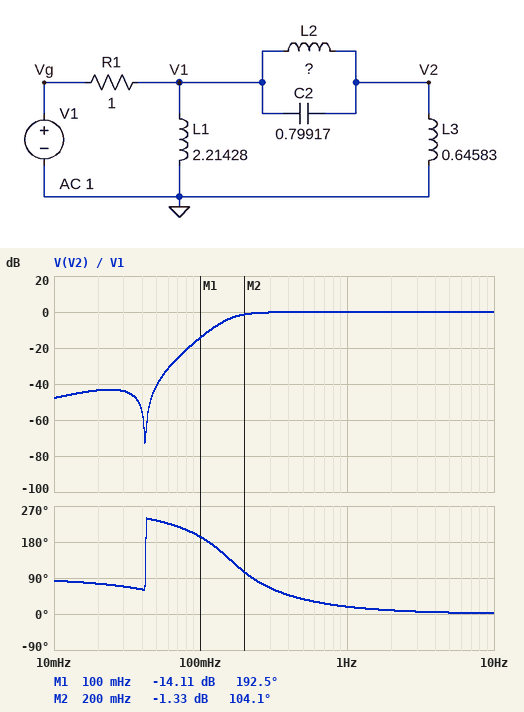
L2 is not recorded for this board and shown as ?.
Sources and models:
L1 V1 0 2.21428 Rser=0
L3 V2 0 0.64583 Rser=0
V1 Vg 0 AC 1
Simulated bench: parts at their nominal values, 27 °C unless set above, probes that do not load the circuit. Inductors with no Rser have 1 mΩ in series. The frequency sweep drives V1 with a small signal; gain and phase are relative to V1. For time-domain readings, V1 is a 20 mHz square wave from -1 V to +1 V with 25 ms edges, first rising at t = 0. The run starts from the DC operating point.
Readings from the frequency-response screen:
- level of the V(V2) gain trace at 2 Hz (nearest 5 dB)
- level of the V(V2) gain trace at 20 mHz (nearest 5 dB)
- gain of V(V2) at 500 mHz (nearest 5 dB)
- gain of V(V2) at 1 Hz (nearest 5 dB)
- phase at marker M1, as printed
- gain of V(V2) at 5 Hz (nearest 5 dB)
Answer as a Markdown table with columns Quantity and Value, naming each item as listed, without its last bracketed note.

| Quantity | Value |
|---|---|
| level of the V(V2) gain trace at 2 Hz | 0 dB |
| level of the V(V2) gain trace at 20 mHz | -45 dB |
| gain of V(V2) at 500 mHz | 0 dB |
| gain of V(V2) at 1 Hz | 0 dB |
| phase at marker M1, as printed | 192.5 deg |
| gain of V(V2) at 5 Hz | 0 dB |
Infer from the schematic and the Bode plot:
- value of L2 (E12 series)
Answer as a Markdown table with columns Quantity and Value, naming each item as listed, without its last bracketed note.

| Quantity | Value |
|---|---|
| value of L2 | 18 H |
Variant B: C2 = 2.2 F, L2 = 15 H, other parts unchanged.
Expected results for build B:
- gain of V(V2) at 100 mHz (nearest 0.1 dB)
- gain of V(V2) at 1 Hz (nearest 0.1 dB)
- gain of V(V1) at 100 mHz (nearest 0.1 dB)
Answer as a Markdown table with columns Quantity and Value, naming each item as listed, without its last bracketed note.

| Quantity | Value |
|---|---|
| gain of V(V2) at 100 mHz | -6.1 dB |
| gain of V(V2) at 1 Hz | -0.3 dB |
| gain of V(V1) at 100 mHz | -6.7 dB |
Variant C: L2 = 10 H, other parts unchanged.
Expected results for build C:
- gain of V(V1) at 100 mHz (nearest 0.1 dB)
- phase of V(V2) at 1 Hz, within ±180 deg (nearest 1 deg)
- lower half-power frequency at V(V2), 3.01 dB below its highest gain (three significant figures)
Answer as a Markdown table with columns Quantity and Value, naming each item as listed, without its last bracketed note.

| Quantity | Value |
|---|---|
| gain of V(V1) at 100 mHz | -0.4 dB |
| phase of V(V2) at 1 Hz, within ±180 deg | 18 deg |
| lower half-power frequency at V(V2), 3.01 dB below its highest gain | 169 mHz |
